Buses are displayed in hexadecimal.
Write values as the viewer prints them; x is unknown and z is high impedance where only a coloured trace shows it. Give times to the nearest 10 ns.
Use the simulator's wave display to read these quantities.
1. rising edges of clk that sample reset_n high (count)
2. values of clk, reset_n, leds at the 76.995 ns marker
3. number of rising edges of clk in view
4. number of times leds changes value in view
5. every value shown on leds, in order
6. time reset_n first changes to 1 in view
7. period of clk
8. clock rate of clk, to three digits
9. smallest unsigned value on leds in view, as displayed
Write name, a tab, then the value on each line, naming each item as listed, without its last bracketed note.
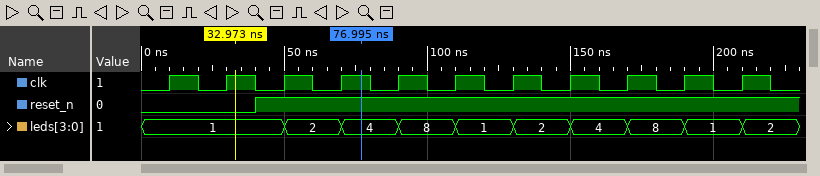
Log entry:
rising edges of clk that sample reset_n high	9
values of clk, reset_n, leds at the 76.995 ns marker	clk=1, reset_n=1, leds=4
number of rising edges of clk in view	11
number of times leds changes value in view	9
every value shown on leds, in order	1, 2, 4, 8, 1, 2, 4, 8, 1, 2
time reset_n first changes to 1 in view	40 ns
period of clk	20 ns
clock rate of clk, to three digits	50.0 MHz
smallest unsigned value on leds in view, as displayed	1
